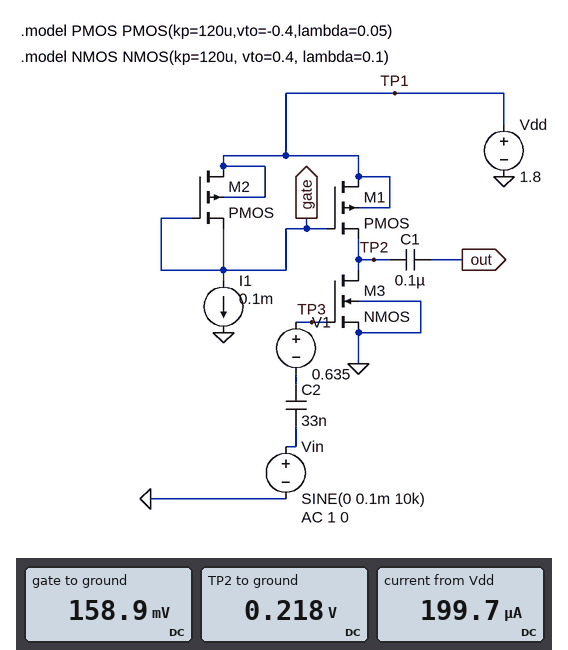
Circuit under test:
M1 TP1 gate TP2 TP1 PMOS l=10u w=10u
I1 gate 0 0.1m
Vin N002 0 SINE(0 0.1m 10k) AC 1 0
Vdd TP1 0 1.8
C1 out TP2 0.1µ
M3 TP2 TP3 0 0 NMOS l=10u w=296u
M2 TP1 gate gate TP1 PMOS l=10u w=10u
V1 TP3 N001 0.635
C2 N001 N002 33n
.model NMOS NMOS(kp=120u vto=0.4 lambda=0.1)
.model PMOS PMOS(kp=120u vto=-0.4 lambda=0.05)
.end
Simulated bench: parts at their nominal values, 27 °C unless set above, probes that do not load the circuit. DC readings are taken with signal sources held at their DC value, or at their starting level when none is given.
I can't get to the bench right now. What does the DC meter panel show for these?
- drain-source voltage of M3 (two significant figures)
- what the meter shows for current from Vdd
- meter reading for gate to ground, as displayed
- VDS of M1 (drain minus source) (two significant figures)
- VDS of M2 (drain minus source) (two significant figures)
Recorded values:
220 mV
199.7 µA
158.9 mV
1.6 V
1.6 V
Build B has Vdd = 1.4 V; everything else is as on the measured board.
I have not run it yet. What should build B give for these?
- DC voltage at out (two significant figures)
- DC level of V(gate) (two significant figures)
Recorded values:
200 mV
-240 mV
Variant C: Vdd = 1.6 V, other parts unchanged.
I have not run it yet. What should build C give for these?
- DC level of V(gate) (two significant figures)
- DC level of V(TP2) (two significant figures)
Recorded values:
-41 mV
210 mV
